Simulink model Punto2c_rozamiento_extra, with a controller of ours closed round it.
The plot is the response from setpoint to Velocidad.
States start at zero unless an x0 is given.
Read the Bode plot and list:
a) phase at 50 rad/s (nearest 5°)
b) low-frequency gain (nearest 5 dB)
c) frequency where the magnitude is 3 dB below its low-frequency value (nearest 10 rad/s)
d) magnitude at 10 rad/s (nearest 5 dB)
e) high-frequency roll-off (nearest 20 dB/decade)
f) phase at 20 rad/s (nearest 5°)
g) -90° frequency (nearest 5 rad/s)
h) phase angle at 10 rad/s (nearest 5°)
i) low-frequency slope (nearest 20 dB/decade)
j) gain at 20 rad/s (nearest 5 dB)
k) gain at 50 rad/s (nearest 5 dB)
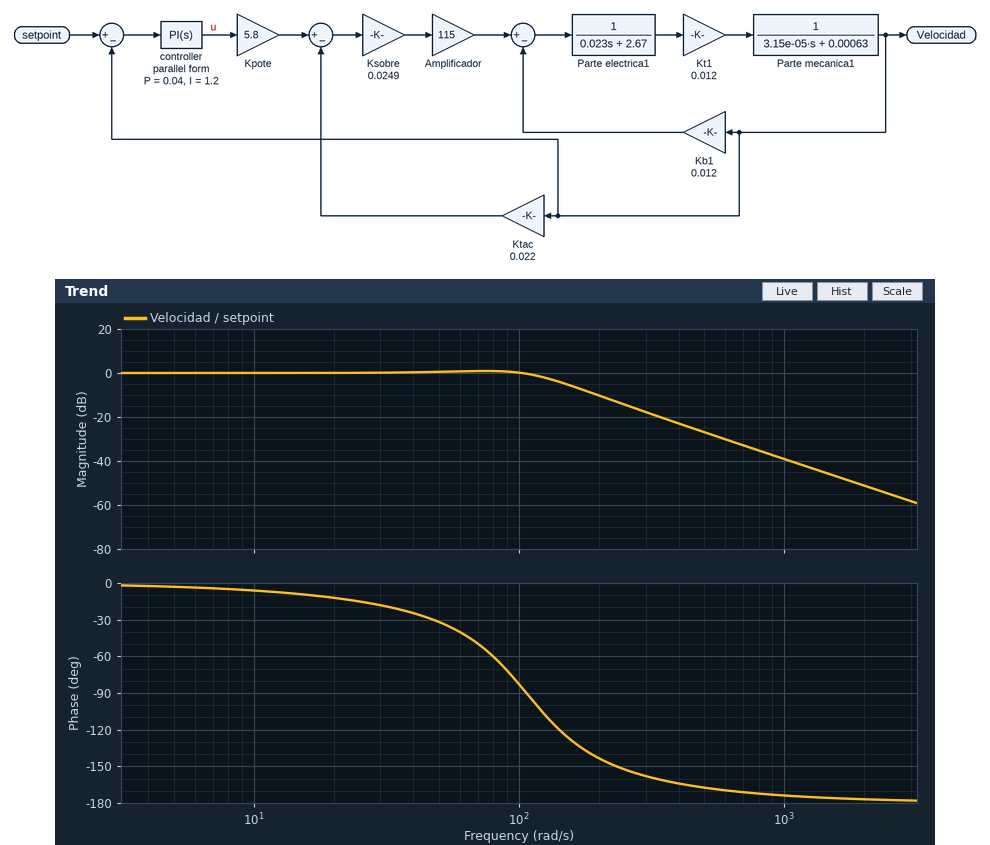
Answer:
-30°
0 dB
130 rad/s
0 dB
-40 dB/decade
-10°
105 rad/s
-5°
0 dB/decade
0 dB
0 dB
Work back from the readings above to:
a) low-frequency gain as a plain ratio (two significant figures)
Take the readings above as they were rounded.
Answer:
1.0
